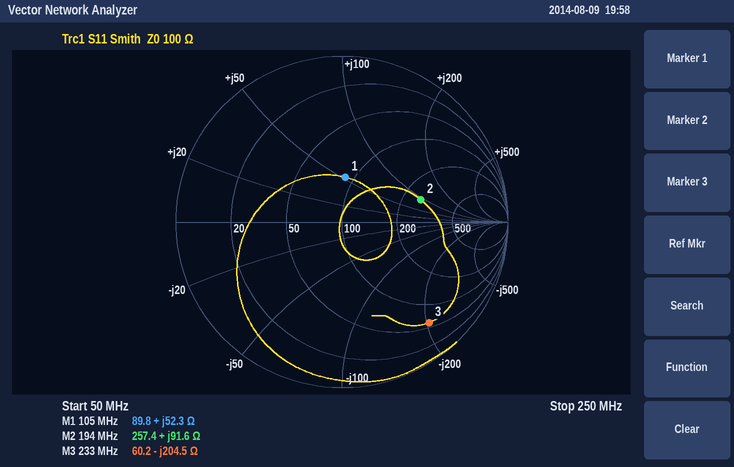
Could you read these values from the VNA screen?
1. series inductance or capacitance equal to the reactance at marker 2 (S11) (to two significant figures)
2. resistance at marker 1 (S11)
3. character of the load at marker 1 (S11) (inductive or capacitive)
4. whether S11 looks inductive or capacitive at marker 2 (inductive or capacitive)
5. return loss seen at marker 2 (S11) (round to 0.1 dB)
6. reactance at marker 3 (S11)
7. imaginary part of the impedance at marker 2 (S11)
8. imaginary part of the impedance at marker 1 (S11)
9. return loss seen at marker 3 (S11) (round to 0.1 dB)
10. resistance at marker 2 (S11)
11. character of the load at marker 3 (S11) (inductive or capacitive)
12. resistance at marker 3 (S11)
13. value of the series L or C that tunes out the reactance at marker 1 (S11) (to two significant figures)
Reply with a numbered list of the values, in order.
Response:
1. 75 nH
2. 89.8 Ω
3. inductive
4. inductive
5. 6.1 dB
6. -204.5 Ω
7. +91.6 Ω
8. +52.3 Ω
9. 1.9 dB
10. 257.4 Ω
11. capacitive
12. 60.2 Ω
13. 29 pF
